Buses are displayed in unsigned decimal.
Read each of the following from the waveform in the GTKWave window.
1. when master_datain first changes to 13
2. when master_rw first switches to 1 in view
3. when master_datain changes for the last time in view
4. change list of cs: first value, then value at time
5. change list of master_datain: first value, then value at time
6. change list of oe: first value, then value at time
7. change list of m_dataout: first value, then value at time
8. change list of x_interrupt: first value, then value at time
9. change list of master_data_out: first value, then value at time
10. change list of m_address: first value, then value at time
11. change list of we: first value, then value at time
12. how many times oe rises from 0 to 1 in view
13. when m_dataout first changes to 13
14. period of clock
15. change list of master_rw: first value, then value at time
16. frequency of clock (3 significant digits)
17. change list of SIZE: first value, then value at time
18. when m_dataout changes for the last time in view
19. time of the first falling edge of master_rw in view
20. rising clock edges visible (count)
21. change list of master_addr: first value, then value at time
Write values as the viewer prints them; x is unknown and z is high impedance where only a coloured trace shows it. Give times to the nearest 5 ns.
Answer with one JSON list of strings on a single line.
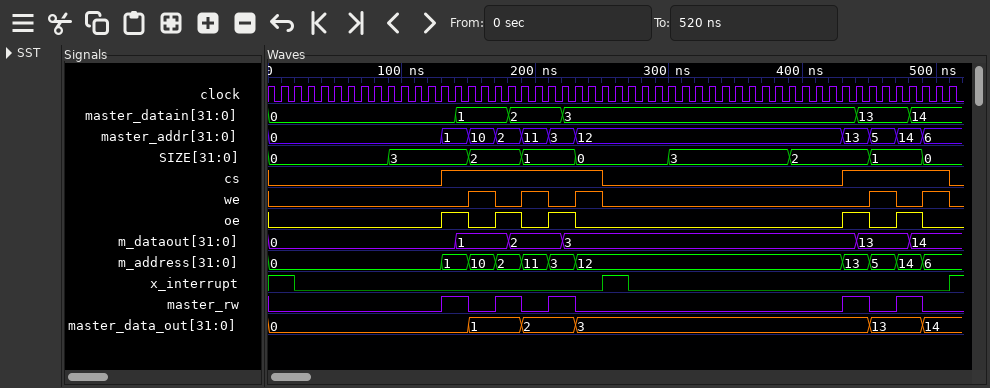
["440 ns", "130 ns", "480 ns", "0, 1 at 130 ns, 0 at 250 ns, 1 at 430 ns, 0 at 510 ns", "0, 1 at 140 ns, 2 at 180 ns, 3 at 220 ns, 13 at 440 ns, 14 at 480 ns", "0, 1 at 130 ns, 0 at 150 ns, 1 at 170 ns, 0 at 190 ns, 1 at 210 ns, 0 at 230 ns, 1 at 430 ns, 0 at 450 ns, 1 at 470 ns, 0 at 490 ns", "0, 1 at 140 ns, 2 at 180 ns, 3 at 220 ns, 13 at 440 ns, 14 at 480 ns", "1, 0 at 20 ns, 1 at 250 ns, 0 at 270 ns, 1 at 510 ns", "0, 1 at 150 ns, 2 at 190 ns, 3 at 230 ns, 13 at 450 ns, 14 at 490 ns", "0, 1 at 130 ns, 10 at 150 ns, 2 at 170 ns, 11 at 190 ns, 3 at 210 ns, 12 at 230 ns, 13 at 430 ns, 5 at 450 ns, 14 at 470 ns, 6 at 490 ns", "0, 1 at 150 ns, 0 at 170 ns, 1 at 190 ns, 0 at 210 ns, 1 at 230 ns, 0 at 250 ns, 1 at 450 ns, 0 at 470 ns, 1 at 490 ns, 0 at 510 ns", "5", "440 ns", "10 ns", "0, 1 at 130 ns, 0 at 150 ns, 1 at 170 ns, 0 at 190 ns, 1 at 210 ns, 0 at 230 ns, 1 at 430 ns, 0 at 450 ns, 1 at 470 ns, 0 at 490 ns", "100 MHz", "0, 3 at 90 ns, 2 at 150 ns, 1 at 190 ns, 0 at 230 ns, 3 at 300 ns, 2 at 390 ns, 1 at 450 ns, 0 at 490 ns", "480 ns", "150 ns", "51", "0, 1 at 130 ns, 10 at 150 ns, 2 at 170 ns, 11 at 190 ns, 3 at 210 ns, 12 at 230 ns, 13 at 430 ns, 5 at 450 ns, 14 at 470 ns, 6 at 490 ns"]
